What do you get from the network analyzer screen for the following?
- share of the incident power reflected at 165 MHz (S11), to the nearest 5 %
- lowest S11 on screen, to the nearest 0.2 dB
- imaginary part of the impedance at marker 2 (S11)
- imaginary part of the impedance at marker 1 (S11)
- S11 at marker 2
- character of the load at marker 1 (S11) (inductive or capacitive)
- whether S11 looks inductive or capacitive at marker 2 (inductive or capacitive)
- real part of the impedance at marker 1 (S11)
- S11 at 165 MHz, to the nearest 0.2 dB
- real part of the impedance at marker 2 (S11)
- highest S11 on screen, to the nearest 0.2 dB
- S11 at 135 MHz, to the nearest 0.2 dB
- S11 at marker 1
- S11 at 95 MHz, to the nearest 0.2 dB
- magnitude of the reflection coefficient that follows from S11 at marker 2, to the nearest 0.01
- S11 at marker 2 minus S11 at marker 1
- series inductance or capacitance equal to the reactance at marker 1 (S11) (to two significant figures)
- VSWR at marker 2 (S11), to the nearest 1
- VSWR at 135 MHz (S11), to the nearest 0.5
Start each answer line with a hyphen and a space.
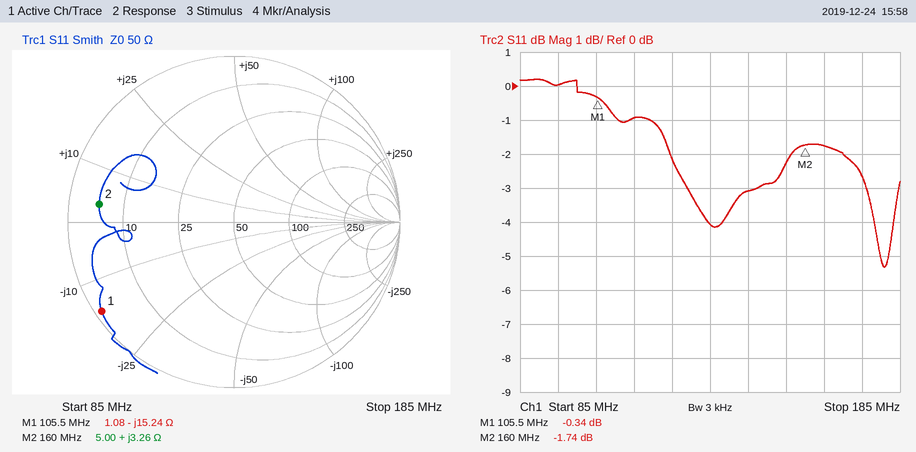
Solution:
- 65 %
- -5.4 dB
- +3.26 Ω
- -15.24 Ω
- -1.74 dB
- capacitive
- inductive
- 1.08 Ω
- -1.8 dB
- 5.00 Ω
- 0.2 dB
- -4.0 dB
- -0.34 dB
- 0.0 dB
- 0.82
- -1.40 dB
- 99 pF
- 10
- 4.5
